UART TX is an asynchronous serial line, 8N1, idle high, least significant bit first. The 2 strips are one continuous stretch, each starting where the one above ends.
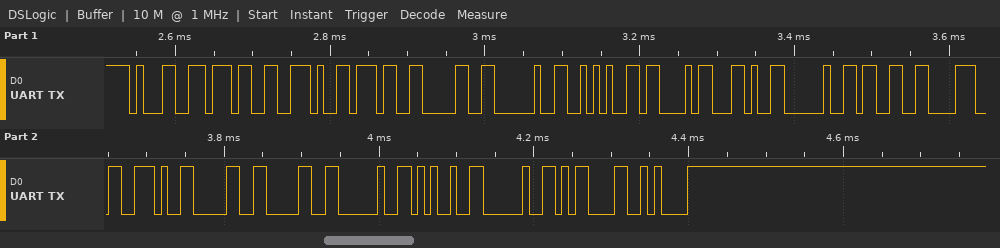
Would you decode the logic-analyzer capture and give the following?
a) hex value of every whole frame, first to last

31 37 2E 37 30 20 2A 43 2C 20 33 38 2E 30 30 20 25 20 0D 0A
